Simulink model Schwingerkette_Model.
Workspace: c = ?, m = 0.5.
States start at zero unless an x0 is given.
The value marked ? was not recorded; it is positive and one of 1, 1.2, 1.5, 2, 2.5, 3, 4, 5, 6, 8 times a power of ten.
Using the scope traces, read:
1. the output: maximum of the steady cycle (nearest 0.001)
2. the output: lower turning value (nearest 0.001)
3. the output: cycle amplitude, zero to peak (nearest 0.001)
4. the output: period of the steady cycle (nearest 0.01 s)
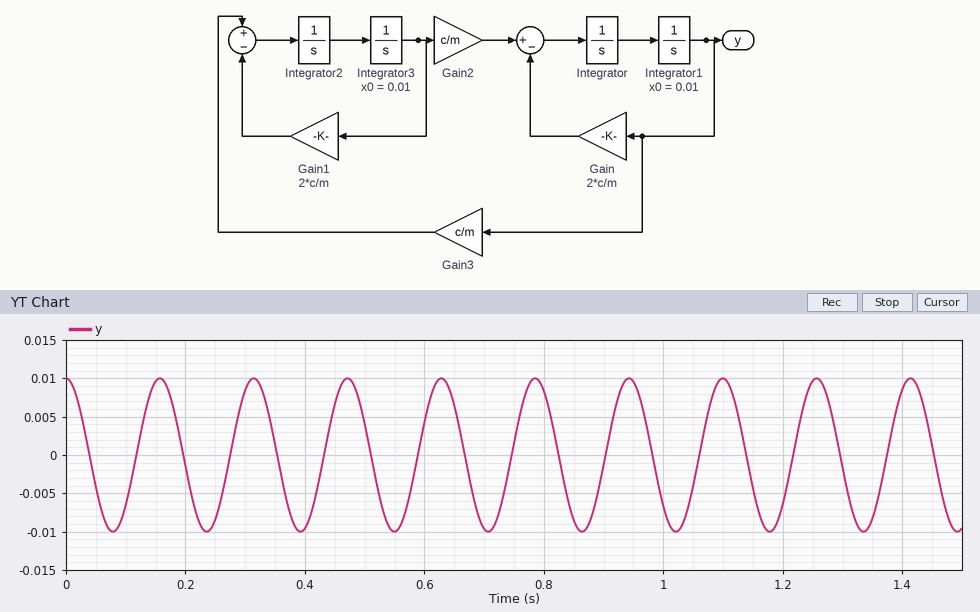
0.010
-0.010
0.010
0.16 s
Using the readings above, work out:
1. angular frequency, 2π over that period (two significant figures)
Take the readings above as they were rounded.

39 rad/s
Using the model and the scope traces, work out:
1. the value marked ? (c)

800
